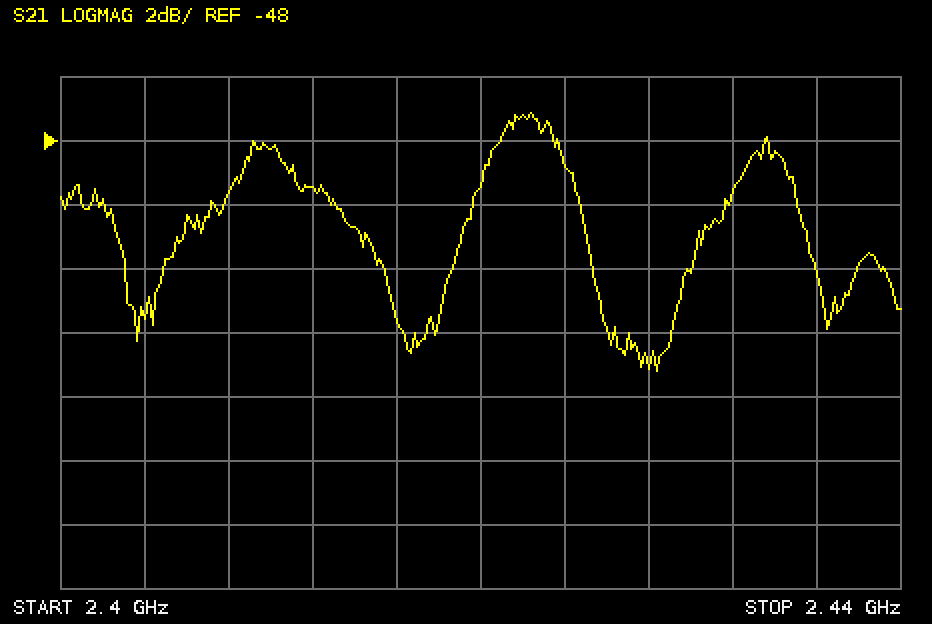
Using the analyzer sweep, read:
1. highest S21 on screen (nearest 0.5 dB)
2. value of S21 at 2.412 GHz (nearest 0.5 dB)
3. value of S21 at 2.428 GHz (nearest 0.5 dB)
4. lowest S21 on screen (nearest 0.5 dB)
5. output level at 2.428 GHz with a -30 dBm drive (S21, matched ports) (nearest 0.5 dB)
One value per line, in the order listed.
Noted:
-47.0 dB
-49.5 dB
-55.0 dB
-55.0 dB
-85.0 dBm
